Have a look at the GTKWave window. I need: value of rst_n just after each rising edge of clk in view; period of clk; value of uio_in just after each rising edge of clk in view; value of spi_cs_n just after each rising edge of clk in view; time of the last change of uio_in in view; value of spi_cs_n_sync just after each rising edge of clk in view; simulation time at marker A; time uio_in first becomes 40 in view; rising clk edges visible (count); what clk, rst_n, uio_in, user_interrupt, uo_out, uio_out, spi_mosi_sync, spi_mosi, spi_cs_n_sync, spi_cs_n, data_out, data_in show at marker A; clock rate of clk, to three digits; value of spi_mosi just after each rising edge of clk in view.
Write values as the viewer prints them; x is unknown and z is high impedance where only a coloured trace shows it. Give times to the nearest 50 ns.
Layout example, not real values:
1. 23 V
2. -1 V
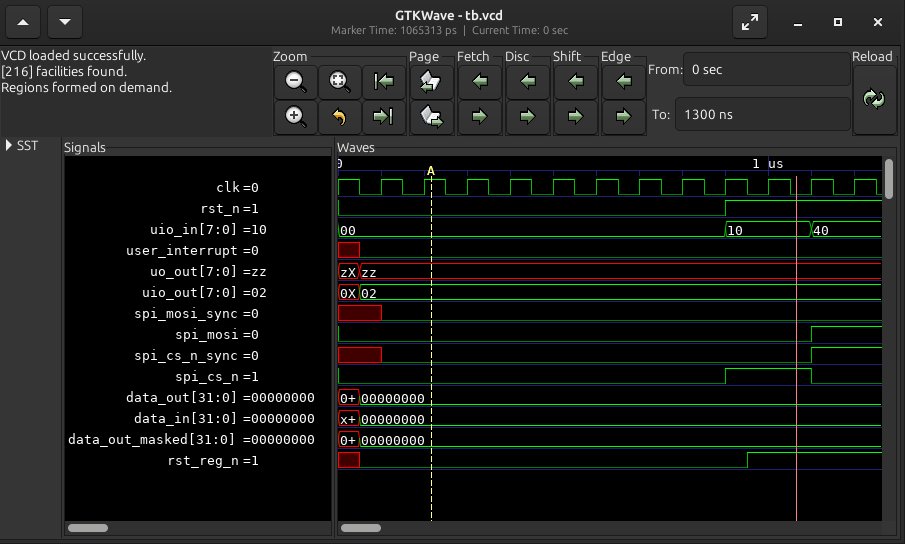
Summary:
1. 0 0 0 0 0 0 0 0 1 1 1 1
2. 100 ns
3. 00, 00, 00, 00, 00, 00, 00, 00, 10, 10, 40, 40
4. 0 0 0 0 0 0 0 0 1 1 0 0
5. 1100 ns
6. 0 0 0 0 0 0 0 0 0 0 1 1
7. 200 ns
8. 1100 ns
9. 12
10. clk=1, rst_n=0, uio_in=00, user_interrupt=0, uo_out=zz, uio_out=02, spi_mosi_sync=0, spi_mosi=0, spi_cs_n_sync=0, spi_cs_n=0, data_out=00000000, data_in=00000000
11. 10.0 MHz
12. 0 0 0 0 0 0 0 0 0 0 1 1
